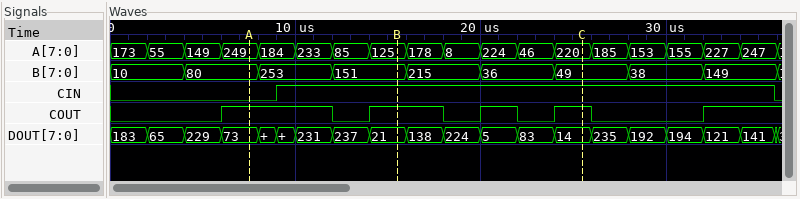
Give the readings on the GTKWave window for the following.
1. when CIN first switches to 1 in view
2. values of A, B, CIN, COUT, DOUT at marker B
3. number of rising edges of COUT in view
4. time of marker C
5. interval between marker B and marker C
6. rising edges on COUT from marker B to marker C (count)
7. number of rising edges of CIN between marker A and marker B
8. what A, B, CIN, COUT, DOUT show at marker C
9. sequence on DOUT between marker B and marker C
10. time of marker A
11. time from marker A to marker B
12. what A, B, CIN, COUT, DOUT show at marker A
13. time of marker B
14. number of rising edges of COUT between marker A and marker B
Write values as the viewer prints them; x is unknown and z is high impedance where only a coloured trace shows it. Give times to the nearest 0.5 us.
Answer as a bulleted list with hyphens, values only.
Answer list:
- 9 us
- A=125, B=151, CIN=1, COUT=1, DOUT=21
- 5
- 25.5 us
- 10 us
- 2
- 1
- A=220, B=49, CIN=1, COUT=1, DOUT=14
- 21, 138, 224, 5, 83, 14
- 7.5 us
- 8 us
- A=249, B=80, CIN=0, COUT=1, DOUT=73
- 15.5 us
- 1
